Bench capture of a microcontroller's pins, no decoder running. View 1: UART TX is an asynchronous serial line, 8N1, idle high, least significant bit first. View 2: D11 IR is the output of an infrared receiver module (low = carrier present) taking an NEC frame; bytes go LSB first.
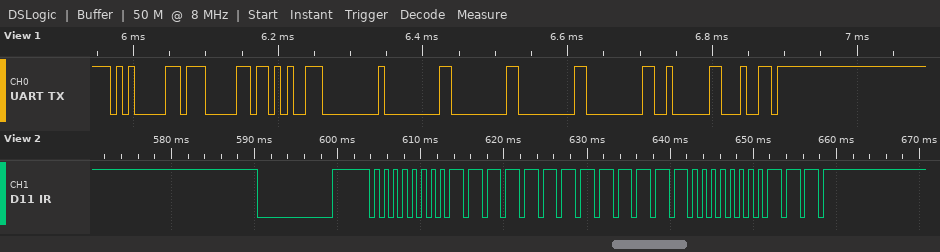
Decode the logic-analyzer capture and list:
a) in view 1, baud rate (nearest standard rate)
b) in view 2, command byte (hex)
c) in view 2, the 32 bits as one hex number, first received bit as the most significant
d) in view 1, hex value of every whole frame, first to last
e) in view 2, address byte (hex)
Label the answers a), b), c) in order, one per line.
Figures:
a) 115200 baud
b) 0x1F
c) 0x00FFF807
d) 0x05 0x07 0x2B 0x00 0x00 0x00 0x00 0x00 0x02 0x64
e) 0x00
